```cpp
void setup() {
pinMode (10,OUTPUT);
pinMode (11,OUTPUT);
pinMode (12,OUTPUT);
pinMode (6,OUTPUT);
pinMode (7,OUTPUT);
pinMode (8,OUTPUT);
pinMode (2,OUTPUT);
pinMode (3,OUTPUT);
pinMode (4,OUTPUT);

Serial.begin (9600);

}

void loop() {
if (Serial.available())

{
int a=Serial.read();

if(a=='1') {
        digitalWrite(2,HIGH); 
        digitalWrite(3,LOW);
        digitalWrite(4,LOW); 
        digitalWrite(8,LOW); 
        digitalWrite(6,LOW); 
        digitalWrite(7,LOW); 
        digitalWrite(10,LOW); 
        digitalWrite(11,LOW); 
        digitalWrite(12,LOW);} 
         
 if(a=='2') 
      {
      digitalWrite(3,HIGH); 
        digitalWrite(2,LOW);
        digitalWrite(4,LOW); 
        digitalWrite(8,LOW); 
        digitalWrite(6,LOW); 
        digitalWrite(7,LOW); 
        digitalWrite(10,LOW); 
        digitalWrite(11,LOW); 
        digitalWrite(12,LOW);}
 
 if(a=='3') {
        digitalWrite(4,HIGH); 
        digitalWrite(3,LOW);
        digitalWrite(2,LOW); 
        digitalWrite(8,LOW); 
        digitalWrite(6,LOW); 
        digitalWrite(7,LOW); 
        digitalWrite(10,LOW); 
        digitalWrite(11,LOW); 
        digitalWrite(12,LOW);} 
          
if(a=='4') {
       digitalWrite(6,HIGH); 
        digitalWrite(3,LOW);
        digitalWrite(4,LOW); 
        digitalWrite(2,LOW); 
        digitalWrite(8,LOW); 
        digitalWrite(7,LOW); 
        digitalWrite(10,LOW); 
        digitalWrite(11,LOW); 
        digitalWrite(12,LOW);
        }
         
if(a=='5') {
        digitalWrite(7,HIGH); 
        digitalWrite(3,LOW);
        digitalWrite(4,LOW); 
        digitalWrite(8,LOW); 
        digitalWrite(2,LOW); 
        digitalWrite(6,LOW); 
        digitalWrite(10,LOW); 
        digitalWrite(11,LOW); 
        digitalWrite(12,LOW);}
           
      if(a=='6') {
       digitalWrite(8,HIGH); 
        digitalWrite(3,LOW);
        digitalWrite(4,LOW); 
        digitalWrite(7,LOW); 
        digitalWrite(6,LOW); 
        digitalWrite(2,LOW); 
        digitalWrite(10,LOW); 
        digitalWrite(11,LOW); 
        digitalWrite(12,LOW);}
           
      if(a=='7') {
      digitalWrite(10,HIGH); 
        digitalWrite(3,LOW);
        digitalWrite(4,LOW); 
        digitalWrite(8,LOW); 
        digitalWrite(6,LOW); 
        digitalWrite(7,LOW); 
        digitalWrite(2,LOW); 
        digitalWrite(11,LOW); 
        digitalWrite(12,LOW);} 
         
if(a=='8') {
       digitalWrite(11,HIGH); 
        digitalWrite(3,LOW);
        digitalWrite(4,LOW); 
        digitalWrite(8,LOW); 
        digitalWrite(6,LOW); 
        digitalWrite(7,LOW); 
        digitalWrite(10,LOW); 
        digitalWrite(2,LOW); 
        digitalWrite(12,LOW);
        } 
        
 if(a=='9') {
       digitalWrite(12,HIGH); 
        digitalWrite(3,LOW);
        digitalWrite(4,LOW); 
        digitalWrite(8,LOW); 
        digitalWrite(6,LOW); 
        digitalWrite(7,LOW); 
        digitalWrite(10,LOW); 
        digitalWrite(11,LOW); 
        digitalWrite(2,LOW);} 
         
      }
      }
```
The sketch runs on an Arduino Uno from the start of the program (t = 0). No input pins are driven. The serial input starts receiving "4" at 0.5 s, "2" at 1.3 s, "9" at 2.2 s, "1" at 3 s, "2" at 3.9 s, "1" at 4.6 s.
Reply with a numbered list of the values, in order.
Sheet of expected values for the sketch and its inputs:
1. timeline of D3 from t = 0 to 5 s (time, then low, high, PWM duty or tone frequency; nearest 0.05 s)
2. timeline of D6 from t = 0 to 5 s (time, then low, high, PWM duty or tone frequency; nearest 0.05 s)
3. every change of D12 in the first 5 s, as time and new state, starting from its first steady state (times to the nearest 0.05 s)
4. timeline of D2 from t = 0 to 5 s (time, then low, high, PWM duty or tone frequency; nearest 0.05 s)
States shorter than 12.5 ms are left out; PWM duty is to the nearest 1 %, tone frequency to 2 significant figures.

1. 0 s low; 1.3 s high; 2.2 s low; 3.9 s high; 4.6 s low
2. 0 s low; 0.5 s high; 1.3 s low
3. 0 s low; 2.2 s high; 3 s low
4. 0 s low; 3 s high; 3.9 s low; 4.6 s high
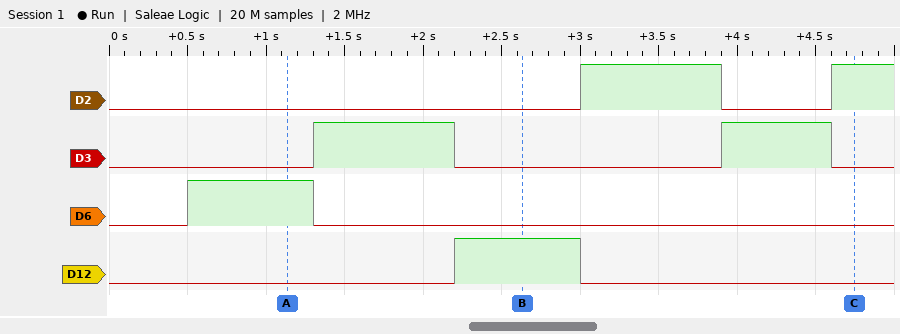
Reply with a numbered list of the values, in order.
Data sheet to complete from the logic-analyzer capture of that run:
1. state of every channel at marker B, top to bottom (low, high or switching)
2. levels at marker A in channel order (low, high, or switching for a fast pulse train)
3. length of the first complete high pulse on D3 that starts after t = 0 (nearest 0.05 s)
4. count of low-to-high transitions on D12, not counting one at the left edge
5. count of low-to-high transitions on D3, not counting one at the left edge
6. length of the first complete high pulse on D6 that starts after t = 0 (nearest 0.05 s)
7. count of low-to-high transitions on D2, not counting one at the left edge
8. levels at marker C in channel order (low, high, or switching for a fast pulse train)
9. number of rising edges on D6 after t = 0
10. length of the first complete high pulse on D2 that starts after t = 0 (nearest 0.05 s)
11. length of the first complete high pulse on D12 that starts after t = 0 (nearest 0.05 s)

1. D2 low, D3 low, D6 low, D12 high
2. D2 low, D3 low, D6 high, D12 low
3. 0.90 s
4. 1
5. 2
6. 0.80 s
7. 2
8. D2 high, D3 low, D6 low, D12 low
9. 1
10. 0.90 s
11. 0.80 s
